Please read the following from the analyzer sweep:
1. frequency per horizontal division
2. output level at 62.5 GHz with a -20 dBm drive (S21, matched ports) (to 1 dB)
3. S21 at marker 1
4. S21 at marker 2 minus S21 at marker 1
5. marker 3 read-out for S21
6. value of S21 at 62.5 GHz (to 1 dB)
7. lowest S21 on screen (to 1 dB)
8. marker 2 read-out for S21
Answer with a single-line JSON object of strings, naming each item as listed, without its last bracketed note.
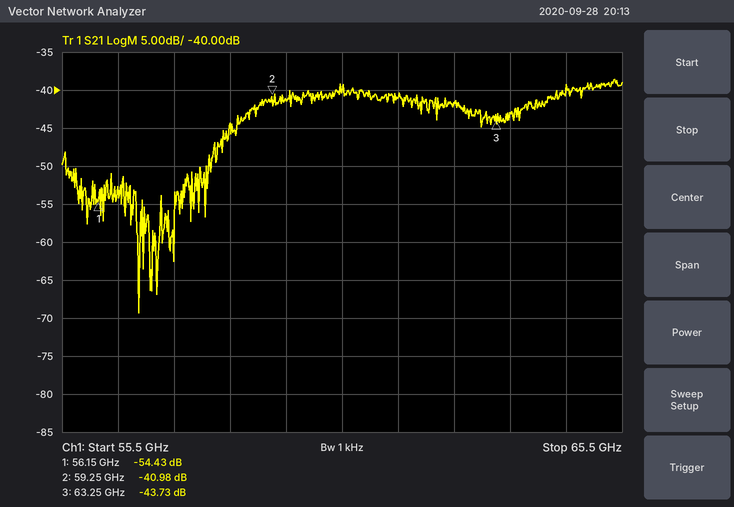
{"frequency per horizontal division": "1 GHz", "output level at 62.5 GHz with a -20 dBm drive (S21, matched ports)": "-62 dBm", "S21 at marker 1": "-54.43 dB", "S21 at marker 2 minus S21 at marker 1": "13.45 dB", "marker 3 read-out for S21": "-43.73 dB", "value of S21 at 62.5 GHz": "-42 dB", "lowest S21 on screen": "-69 dB", "marker 2 read-out for S21": "-40.98 dB"}
